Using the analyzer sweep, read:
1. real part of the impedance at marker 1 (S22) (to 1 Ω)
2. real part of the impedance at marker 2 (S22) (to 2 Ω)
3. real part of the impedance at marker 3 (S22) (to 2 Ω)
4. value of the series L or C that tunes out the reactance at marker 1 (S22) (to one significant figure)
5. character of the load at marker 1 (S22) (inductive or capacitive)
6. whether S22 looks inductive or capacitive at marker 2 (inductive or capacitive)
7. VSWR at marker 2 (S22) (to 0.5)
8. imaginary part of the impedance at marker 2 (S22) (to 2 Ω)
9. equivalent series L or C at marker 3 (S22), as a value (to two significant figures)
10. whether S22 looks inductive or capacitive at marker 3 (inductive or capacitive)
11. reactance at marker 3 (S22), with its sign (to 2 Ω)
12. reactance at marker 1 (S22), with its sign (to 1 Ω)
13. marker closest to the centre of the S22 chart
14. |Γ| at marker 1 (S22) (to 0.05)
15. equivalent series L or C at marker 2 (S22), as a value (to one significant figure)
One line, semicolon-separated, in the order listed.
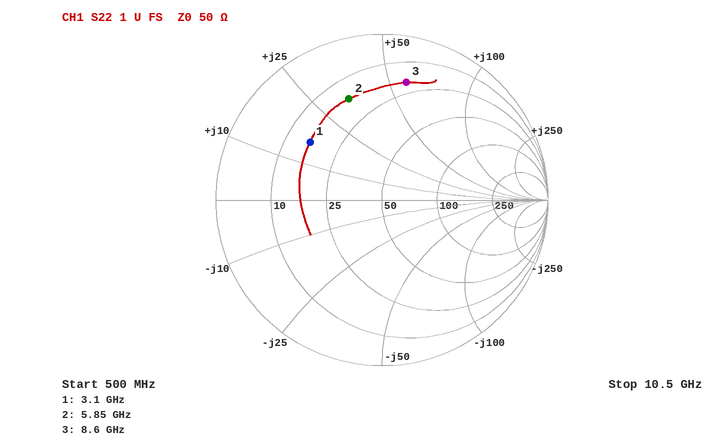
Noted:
16 Ω; 16 Ω; 20 Ω; 3 pF; inductive; inductive; 4.5; +34 Ω; 1.1 nH; inductive; +58 Ω; +16 Ω; marker 1; 0.55; 900 pH
